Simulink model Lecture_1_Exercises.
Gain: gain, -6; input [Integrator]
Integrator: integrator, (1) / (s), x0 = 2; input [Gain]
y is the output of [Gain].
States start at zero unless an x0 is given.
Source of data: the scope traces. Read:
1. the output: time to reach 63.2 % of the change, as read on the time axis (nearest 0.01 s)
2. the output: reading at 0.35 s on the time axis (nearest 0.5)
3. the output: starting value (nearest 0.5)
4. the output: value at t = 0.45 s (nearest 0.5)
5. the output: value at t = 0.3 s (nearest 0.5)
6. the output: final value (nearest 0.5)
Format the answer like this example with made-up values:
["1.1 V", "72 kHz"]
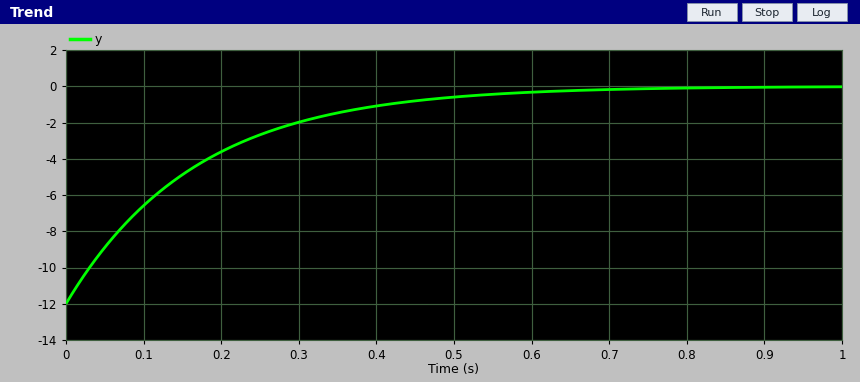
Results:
["0.17 s", "-1.5", "-12.0", "-1.0", "-2.0", "0.0"]
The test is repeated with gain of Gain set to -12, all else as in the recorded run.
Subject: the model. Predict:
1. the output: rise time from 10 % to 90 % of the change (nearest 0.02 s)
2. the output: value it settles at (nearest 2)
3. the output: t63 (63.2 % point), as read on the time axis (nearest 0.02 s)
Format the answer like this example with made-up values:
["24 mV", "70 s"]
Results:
["0.18 s", "0", "0.08 s"]
